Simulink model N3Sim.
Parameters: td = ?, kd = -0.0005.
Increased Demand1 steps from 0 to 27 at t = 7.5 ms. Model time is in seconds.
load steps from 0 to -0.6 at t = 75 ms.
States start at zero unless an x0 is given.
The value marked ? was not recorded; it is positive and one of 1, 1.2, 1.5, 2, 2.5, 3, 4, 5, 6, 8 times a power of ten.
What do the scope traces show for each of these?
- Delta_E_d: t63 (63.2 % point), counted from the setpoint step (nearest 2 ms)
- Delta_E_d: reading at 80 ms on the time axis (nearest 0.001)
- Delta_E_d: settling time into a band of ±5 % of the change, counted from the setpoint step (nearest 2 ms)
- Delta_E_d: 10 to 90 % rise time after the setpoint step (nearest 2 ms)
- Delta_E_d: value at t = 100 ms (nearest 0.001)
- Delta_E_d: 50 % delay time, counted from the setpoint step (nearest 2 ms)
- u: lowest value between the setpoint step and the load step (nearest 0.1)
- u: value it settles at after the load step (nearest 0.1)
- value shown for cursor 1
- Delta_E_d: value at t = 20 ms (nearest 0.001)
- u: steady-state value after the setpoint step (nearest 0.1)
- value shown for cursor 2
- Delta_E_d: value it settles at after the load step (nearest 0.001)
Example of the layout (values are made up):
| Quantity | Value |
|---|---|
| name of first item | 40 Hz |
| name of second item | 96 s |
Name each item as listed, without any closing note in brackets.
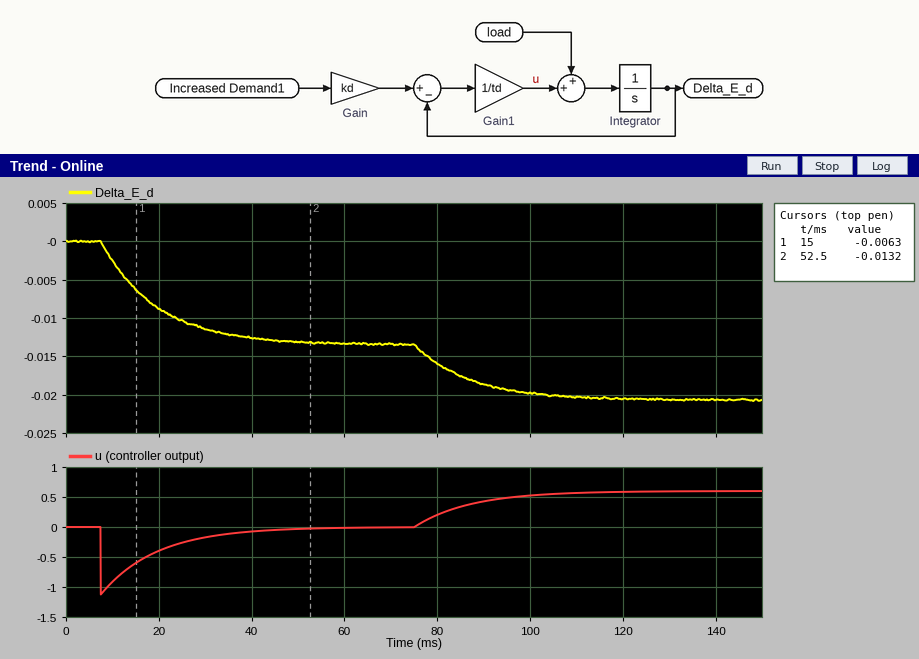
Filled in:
| Quantity | Value |
|---|---|
| Delta_E_d: t63 (63.2 % point), counted from the setpoint step | 12 ms |
| Delta_E_d: reading at 80 ms on the time axis | -0.016 |
| Delta_E_d: settling time into a band of ±5 % of the change, counted from the setpoint step | 36 ms |
| Delta_E_d: 10 to 90 % rise time after the setpoint step | 26 ms |
| Delta_E_d: value at t = 100 ms | -0.020 |
| Delta_E_d: 50 % delay time, counted from the setpoint step | 8 ms |
| u: lowest value between the setpoint step and the load step | -1.1 |
| u: value it settles at after the load step | 0.6 |
| value shown for cursor 1 | -0.0063 |
| Delta_E_d: value at t = 20 ms | -0.009 |
| u: steady-state value after the setpoint step | 0.0 |
| value shown for cursor 2 | -0.0132 |
| Delta_E_d: value it settles at after the load step | -0.021 |
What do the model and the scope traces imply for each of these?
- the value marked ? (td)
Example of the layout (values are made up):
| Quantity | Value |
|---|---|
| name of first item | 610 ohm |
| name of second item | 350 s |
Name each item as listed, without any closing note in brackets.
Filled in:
| Quantity | Value |
|---|---|
| the value marked ? | 0.012 |
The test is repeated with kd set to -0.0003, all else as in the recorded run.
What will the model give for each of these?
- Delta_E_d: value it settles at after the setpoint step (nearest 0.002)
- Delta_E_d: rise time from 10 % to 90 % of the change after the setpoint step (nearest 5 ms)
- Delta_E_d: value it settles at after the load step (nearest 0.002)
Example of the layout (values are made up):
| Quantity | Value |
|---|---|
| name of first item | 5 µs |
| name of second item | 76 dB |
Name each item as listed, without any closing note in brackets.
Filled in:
| Quantity | Value |
|---|---|
| Delta_E_d: value it settles at after the setpoint step | -0.008 |
| Delta_E_d: rise time from 10 % to 90 % of the change after the setpoint step | 25 ms |
| Delta_E_d: value it settles at after the load step | -0.016 |
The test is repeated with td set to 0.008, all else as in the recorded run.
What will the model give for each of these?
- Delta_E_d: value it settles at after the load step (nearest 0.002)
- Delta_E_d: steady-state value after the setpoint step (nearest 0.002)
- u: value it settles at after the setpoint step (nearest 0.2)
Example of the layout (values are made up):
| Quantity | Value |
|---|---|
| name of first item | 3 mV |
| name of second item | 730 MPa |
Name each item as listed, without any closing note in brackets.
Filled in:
| Quantity | Value |
|---|---|
| Delta_E_d: value it settles at after the load step | -0.018 |
| Delta_E_d: steady-state value after the setpoint step | -0.014 |
| u: value it settles at after the setpoint step | 0.0 |
